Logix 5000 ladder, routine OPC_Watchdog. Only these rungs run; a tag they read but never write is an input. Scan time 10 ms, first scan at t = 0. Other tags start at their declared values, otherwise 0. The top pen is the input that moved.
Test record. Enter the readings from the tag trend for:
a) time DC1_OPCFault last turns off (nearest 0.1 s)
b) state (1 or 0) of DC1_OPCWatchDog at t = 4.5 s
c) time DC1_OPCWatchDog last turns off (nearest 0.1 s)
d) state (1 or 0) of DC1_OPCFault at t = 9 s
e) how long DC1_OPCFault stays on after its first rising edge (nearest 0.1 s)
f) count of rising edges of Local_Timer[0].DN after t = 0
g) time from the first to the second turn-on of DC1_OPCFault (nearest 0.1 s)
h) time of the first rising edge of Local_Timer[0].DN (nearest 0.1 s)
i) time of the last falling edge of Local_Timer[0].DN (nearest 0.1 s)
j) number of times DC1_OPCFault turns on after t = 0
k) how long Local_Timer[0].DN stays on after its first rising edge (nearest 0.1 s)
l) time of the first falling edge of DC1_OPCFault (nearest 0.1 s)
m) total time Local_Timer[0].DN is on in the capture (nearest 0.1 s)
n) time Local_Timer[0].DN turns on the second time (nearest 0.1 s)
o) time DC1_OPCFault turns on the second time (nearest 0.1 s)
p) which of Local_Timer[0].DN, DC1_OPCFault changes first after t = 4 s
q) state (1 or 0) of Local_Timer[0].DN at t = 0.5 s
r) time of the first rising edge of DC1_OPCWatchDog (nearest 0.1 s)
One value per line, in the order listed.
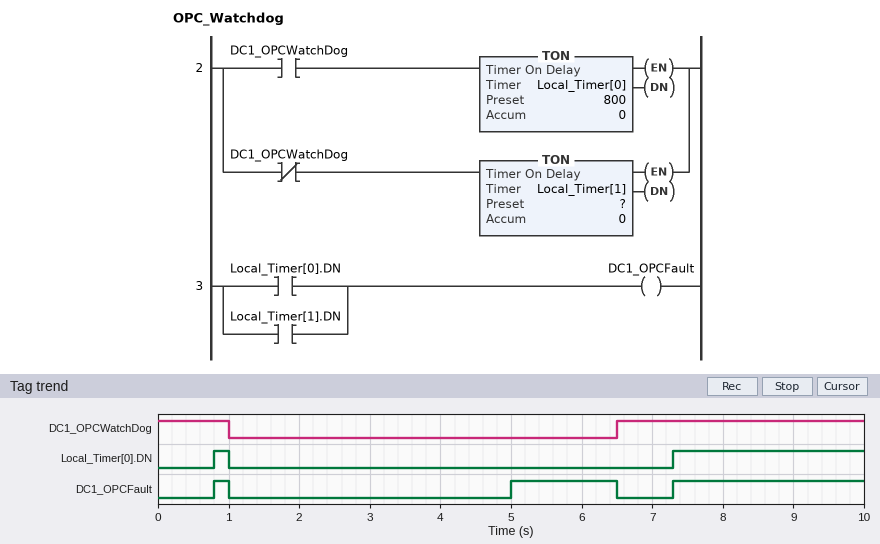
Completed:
6.5 s
0
1.0 s
1
0.2 s
2
4.2 s
0.8 s
1.0 s
3
0.2 s
1.0 s
2.9 s
7.3 s
5.0 s
DC1_OPCFault
0
6.5 s
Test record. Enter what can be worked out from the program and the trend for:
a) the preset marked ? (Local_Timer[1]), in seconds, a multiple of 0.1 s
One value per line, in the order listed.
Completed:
4.0 s
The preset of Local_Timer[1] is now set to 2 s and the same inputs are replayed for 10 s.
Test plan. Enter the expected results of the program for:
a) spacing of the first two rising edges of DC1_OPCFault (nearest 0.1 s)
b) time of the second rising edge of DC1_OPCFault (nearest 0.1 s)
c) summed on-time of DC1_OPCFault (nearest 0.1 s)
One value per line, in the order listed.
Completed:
2.2 s
3.0 s
6.4 s
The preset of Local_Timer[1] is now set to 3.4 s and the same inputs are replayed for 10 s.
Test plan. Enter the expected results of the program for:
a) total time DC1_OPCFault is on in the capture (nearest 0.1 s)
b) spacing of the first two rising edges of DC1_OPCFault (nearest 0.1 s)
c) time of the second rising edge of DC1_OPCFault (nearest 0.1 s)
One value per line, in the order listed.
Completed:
5.0 s
3.6 s
4.4 s
